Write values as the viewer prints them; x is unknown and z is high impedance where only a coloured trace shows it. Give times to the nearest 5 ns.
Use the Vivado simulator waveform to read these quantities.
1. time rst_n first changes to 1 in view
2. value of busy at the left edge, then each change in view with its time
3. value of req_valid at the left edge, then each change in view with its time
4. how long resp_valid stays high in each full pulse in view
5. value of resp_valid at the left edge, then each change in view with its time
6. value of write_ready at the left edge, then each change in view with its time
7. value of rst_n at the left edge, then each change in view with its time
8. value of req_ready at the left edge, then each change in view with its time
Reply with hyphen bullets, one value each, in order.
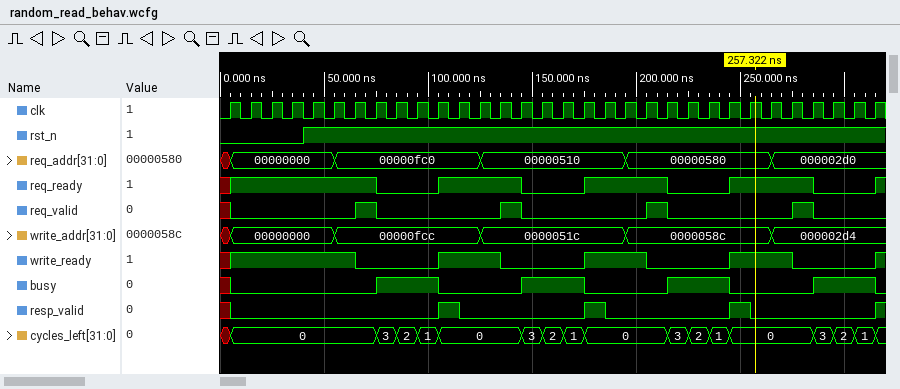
- 40 ns
- x, 0 at 5 ns, 1 at 75 ns, 0 at 105 ns, 1 at 145 ns, 0 at 175 ns, 1 at 215 ns, 0 at 245 ns, 1 at 285 ns, 0 at 315 ns
- x, 0 at 5 ns, 1 at 65 ns, 0 at 75 ns, 1 at 135 ns, 0 at 145 ns, 1 at 205 ns, 0 at 215 ns, 1 at 275 ns, 0 at 285 ns
- 10 ns, 10 ns, 10 ns
- x, 0 at 5 ns, 1 at 105 ns, 0 at 115 ns, 1 at 175 ns, 0 at 185 ns, 1 at 245 ns, 0 at 255 ns, 1 at 315 ns
- x, 1 at 5 ns, 0 at 65 ns, 1 at 105 ns, 0 at 135 ns, 1 at 175 ns, 0 at 205 ns, 1 at 245 ns, 0 at 275 ns, 1 at 315 ns
- 0, 1 at 40 ns
- x, 1 at 5 ns, 0 at 75 ns, 1 at 105 ns, 0 at 145 ns, 1 at 175 ns, 0 at 215 ns, 1 at 245 ns, 0 at 285 ns, 1 at 315 ns
